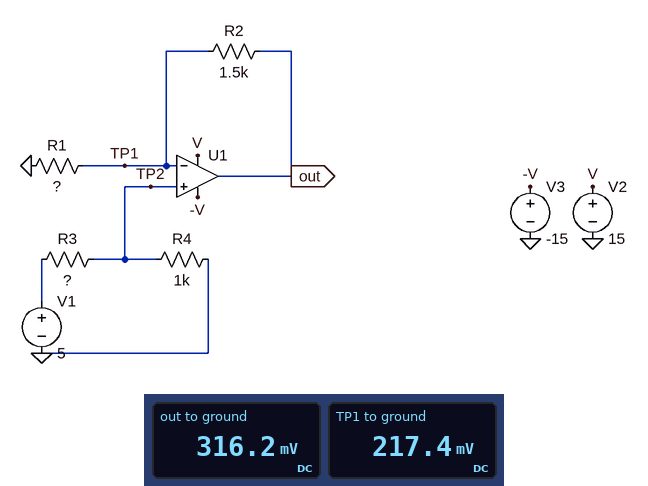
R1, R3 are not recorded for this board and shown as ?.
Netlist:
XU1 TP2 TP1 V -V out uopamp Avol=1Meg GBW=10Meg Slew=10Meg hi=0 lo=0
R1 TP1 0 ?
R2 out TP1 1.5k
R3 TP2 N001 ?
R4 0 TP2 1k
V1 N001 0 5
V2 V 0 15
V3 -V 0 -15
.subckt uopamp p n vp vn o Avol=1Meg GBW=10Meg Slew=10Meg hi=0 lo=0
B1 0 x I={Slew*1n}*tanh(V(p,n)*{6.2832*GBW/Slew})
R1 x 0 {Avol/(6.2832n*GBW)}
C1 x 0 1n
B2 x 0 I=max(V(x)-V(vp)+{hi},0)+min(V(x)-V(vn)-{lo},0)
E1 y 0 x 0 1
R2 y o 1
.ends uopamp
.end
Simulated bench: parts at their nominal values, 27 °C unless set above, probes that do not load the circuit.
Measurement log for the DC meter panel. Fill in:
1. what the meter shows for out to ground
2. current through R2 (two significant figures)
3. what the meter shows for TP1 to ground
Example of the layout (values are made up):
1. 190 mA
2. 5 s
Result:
1. 316.2 mV
2. 66 µA
3. 217.4 mV
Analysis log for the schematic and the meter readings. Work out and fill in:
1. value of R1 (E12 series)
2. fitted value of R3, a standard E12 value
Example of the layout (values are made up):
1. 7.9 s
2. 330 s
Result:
1. 3.3 kΩ
2. 22 kΩ
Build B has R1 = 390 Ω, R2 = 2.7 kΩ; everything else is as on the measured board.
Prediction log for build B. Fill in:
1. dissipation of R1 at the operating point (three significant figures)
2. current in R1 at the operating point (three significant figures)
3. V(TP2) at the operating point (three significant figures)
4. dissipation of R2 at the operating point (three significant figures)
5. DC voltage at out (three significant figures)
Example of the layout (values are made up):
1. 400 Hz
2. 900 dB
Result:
1. 121 µW
2. 557 µA
3. 217 mV
4. 839 µW
5. 1.72 V
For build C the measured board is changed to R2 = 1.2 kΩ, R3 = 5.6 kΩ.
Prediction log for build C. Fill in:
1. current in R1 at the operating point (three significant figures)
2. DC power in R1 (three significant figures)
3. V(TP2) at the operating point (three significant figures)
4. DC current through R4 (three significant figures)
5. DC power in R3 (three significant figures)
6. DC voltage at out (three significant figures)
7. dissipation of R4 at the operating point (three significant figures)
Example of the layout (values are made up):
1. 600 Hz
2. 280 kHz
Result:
1. 230 µA
2. 174 µW
3. 758 mV
4. 758 µA
5. 3.21 mW
6. 1.03 V
7. 574 µW
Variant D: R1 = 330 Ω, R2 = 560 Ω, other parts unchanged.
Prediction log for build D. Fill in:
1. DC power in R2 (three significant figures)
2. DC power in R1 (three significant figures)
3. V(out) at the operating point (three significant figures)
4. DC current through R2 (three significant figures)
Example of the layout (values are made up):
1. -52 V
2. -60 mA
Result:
1. 243 µW
2. 143 µW
3. 586 mV
4. 659 µA
